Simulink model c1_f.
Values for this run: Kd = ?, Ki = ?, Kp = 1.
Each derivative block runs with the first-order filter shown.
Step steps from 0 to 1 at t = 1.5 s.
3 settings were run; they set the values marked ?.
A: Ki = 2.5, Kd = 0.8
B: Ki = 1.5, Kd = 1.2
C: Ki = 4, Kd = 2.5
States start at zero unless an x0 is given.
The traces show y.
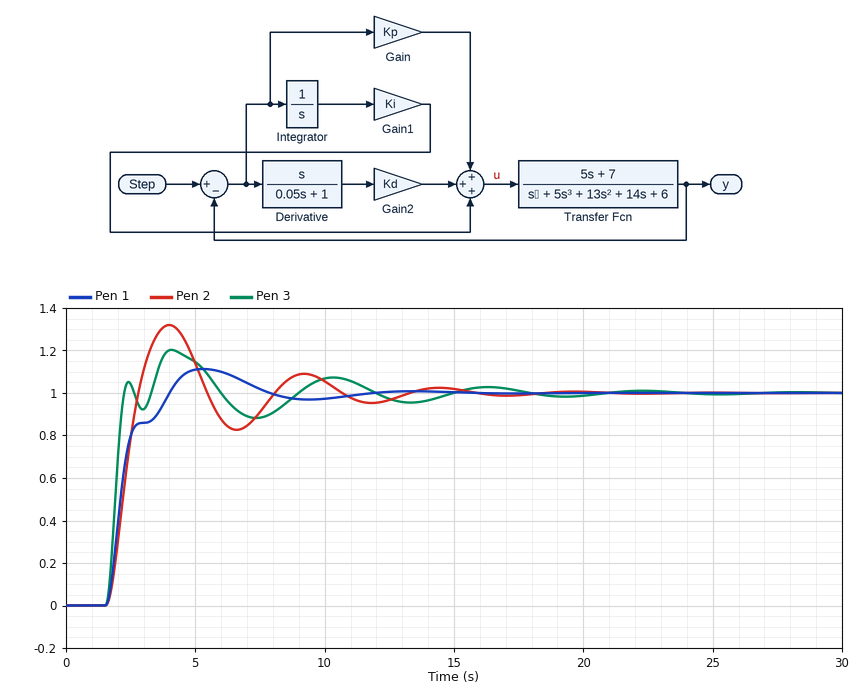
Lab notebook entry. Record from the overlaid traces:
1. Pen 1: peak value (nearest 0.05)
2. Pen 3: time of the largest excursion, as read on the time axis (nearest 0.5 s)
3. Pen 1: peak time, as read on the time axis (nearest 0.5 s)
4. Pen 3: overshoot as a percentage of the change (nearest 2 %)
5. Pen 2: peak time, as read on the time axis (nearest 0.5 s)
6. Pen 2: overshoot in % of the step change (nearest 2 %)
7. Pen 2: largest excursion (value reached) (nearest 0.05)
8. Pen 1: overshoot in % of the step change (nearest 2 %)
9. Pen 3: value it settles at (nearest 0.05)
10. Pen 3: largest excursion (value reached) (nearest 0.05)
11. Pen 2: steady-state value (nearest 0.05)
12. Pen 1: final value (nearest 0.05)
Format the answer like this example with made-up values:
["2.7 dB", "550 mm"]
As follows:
["1.10", "4.0 s", "5.5 s", "20 %", "4.0 s", "32 %", "1.30", "12 %", "1.00", "1.20", "1.00", "1.00"]
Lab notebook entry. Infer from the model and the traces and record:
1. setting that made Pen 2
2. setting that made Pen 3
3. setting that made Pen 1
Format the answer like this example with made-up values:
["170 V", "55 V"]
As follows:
["A", "C", "B"]
